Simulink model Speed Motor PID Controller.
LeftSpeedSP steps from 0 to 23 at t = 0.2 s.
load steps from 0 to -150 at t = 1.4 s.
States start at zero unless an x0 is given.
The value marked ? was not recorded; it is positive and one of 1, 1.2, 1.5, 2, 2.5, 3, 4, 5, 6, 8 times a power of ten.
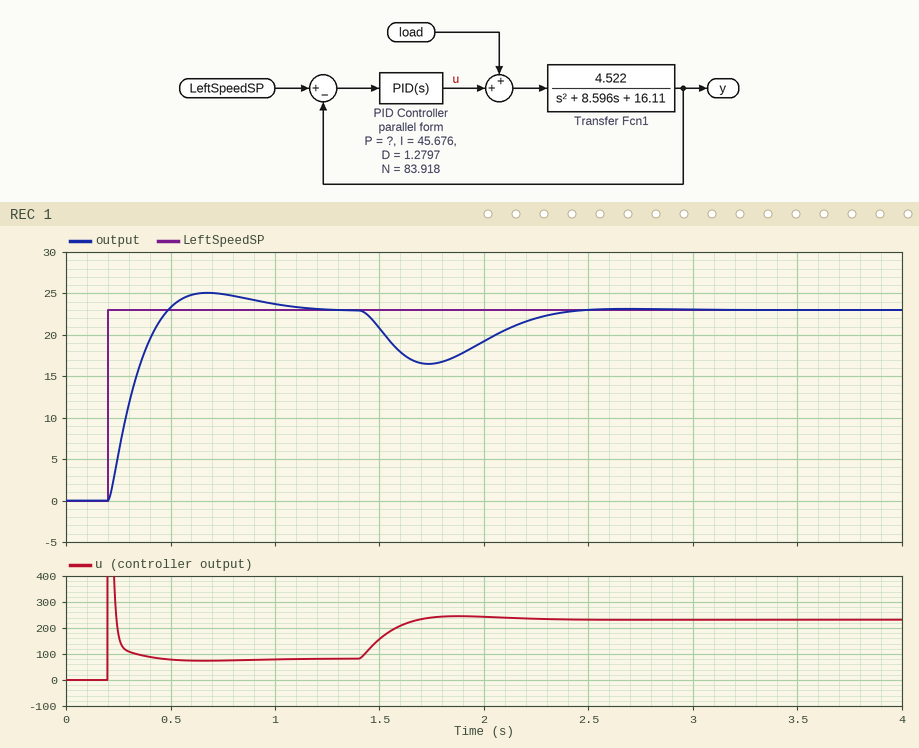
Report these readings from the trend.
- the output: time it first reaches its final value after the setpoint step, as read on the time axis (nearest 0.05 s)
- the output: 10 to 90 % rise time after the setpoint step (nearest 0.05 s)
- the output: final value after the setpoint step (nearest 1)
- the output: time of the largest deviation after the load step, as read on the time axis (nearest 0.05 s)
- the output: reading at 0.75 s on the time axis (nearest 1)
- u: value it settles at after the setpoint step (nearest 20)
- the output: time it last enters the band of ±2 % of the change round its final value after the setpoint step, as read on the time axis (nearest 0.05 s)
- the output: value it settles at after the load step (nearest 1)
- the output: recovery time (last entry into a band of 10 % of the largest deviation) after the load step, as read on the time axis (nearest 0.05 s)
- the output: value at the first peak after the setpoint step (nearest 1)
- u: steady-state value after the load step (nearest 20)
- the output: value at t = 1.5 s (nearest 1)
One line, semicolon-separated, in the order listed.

0.50 s; 0.20 s; 23; 1.75 s; 25; 80; 1.05 s; 23; 2.30 s; 25; 240; 21
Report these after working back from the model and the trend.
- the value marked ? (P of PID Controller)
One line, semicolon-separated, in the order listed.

15
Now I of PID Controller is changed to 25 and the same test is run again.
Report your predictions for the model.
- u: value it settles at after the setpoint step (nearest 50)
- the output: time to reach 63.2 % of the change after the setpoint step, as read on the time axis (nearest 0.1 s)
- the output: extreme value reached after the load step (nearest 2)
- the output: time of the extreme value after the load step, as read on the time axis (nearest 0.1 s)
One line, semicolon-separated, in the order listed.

100; 0.3 s; 16; 1.8 s
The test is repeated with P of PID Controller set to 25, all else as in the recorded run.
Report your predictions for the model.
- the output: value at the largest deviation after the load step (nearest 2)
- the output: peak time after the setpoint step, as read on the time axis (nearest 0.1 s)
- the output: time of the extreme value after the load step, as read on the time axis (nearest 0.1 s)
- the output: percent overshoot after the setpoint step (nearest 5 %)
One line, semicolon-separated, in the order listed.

18; 0.5 s; 1.7 s; 10 %
